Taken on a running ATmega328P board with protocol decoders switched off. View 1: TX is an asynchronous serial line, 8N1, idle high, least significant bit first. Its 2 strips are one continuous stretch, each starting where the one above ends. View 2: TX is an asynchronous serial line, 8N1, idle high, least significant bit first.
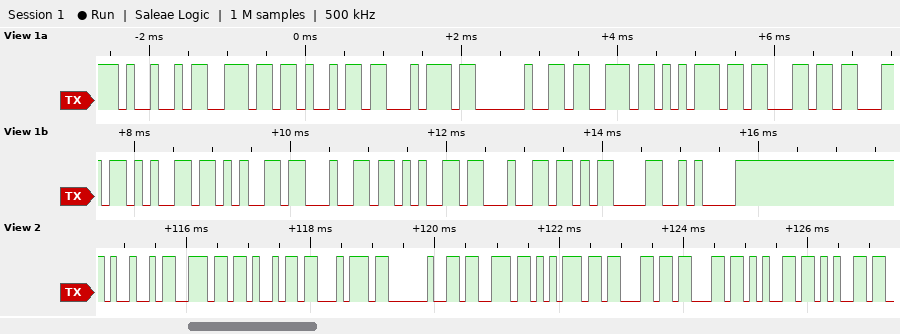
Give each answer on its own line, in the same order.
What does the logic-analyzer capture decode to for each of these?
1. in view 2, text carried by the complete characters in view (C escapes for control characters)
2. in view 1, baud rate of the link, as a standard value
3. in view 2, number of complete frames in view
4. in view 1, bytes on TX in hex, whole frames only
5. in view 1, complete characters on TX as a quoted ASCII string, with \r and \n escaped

"Init succee"
9600 baud
11
49 6E 69 74 20 73 75 63 63 65 65 64 65 64 0D 0A
"Init succeeded\r\n"
